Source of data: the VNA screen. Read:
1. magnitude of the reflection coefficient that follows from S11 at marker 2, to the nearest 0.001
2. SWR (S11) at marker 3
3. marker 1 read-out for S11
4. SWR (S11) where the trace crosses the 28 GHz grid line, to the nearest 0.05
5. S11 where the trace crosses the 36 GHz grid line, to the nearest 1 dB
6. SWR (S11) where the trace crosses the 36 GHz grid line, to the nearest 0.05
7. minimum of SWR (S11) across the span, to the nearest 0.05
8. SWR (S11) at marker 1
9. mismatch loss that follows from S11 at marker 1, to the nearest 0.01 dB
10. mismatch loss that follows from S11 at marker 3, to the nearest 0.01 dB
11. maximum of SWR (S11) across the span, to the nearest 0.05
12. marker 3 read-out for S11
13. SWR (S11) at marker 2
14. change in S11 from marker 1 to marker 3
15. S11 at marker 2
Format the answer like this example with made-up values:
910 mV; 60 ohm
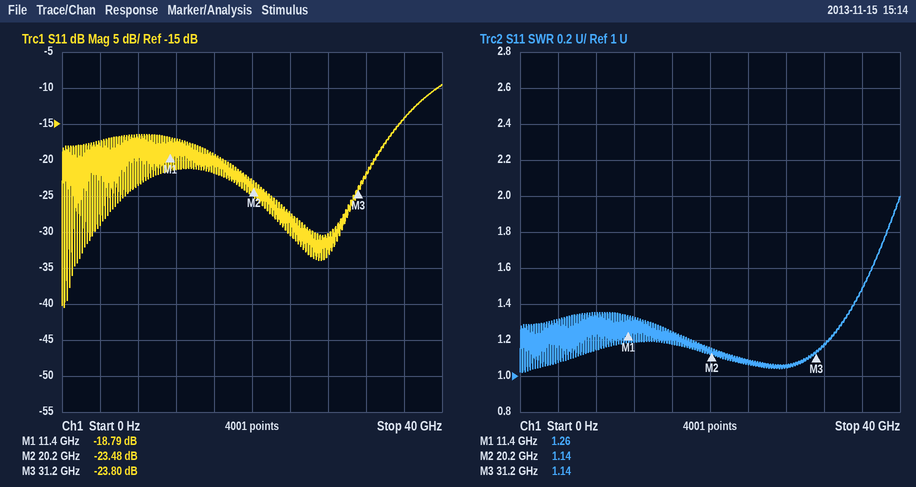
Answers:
0.067; 1.14; -18.79 dB; 1.05; -14 dB; 1.50; 1.00; 1.26; 0.06 dB; 0.02 dB; 2.00; -23.80 dB; 1.14; -5.01 dB; -23.48 dB
